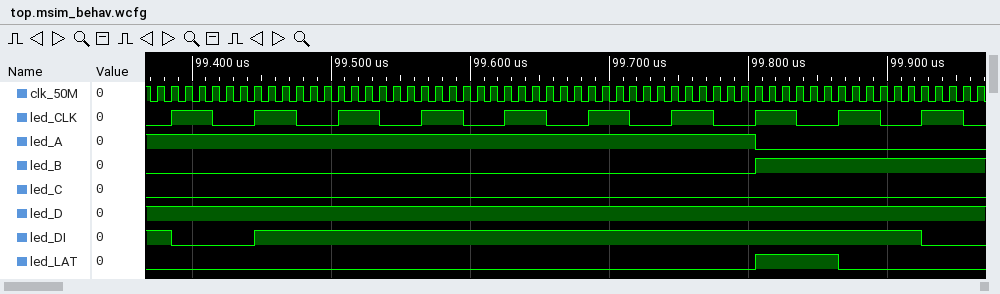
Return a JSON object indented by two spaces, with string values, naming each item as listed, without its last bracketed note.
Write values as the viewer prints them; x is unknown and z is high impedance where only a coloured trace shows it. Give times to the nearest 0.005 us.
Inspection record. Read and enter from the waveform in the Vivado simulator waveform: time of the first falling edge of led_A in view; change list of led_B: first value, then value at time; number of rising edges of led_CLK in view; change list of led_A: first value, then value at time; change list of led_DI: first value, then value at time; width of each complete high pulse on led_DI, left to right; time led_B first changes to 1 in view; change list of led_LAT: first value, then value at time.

{
  "time of the first falling edge of led_A in view": "99.805 us",
  "change list of led_B: first value, then value at time": "0, 1 at 99.805 us",
  "number of rising edges of led_CLK in view": "10",
  "change list of led_A: first value, then value at time": "1, 0 at 99.805 us",
  "change list of led_DI: first value, then value at time": "1, 0 at 99.385 us, 1 at 99.445 us, 0 at 99.925 us",
  "width of each complete high pulse on led_DI, left to right": "0.48 us",
  "time led_B first changes to 1 in view": "99.805 us",
  "change list of led_LAT: first value, then value at time": "0, 1 at 99.805 us, 0 at 99.865 us"
}
